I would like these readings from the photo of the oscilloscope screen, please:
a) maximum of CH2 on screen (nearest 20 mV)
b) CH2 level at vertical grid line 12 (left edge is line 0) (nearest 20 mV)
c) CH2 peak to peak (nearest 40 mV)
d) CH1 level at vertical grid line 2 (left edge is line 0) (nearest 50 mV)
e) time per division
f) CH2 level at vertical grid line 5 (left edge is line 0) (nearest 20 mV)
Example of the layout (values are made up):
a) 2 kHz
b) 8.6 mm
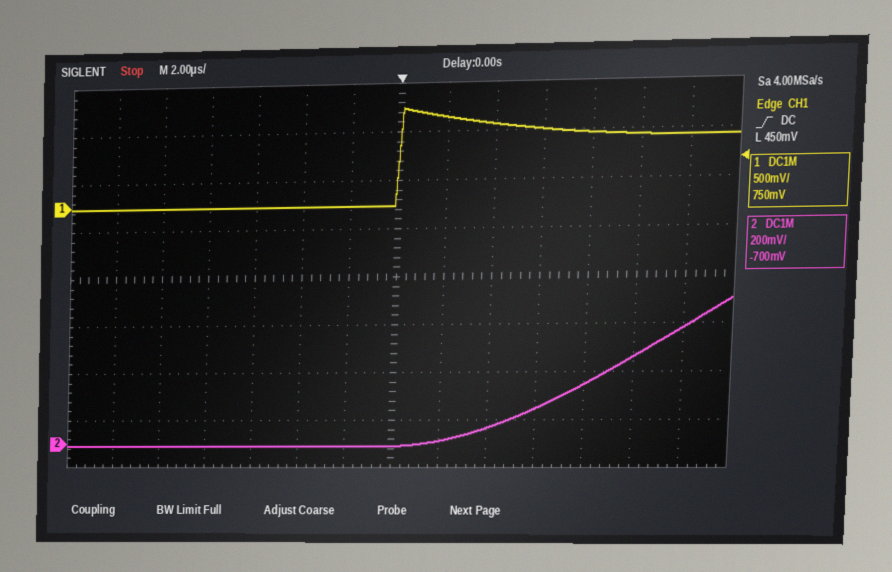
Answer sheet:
a) 600 mV
b) 360 mV
c) 600 mV
d) 0 mV
e) 2 µs
f) 0 mV
